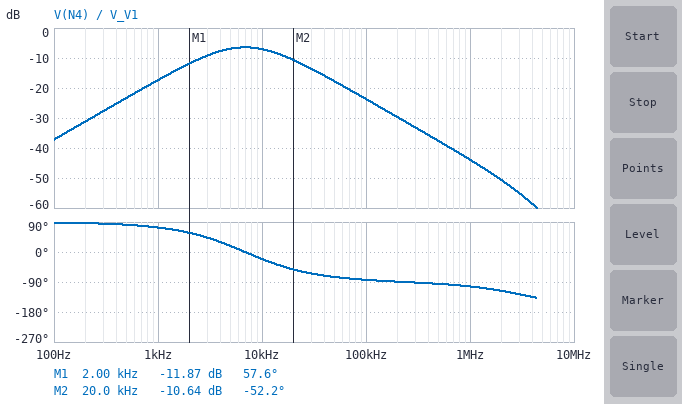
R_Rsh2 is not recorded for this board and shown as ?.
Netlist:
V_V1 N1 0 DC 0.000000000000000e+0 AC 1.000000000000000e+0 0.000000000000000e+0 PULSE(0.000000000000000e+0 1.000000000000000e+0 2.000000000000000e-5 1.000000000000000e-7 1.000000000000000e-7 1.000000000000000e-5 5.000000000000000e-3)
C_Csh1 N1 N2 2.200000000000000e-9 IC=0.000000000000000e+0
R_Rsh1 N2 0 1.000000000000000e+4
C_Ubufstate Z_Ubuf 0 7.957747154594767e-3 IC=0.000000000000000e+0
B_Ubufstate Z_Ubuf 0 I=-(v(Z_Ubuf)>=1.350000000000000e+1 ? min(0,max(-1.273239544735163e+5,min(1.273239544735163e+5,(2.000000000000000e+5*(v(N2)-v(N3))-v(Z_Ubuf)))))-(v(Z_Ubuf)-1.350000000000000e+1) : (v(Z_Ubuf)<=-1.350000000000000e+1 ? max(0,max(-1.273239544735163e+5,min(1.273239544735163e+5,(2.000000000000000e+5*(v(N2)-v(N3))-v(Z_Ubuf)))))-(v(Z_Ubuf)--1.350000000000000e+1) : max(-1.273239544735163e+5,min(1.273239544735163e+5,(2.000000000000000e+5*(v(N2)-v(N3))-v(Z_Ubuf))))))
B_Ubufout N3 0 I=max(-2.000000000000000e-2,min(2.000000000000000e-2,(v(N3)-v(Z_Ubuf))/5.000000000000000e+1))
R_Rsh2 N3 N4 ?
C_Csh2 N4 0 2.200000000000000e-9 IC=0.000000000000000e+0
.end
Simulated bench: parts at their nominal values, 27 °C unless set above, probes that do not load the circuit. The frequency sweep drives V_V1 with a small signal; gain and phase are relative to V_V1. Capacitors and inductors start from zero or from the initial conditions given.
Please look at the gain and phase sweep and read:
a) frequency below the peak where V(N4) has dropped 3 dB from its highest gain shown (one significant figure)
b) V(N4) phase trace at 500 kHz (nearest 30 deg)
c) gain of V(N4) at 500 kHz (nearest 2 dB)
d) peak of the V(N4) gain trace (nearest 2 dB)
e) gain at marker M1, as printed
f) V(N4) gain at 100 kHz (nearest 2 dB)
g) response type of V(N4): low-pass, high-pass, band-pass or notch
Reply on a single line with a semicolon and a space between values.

3 kHz; -90 deg; -38 dB; -6 dB; -11.87 dB; -24 dB; band-pass
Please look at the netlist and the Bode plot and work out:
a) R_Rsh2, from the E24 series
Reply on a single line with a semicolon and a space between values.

11 kΩ
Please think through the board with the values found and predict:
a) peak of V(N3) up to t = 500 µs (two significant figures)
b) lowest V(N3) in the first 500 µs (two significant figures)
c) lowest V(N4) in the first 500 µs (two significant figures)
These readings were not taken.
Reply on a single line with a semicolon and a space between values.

990 mV; -360 mV; -56 mV
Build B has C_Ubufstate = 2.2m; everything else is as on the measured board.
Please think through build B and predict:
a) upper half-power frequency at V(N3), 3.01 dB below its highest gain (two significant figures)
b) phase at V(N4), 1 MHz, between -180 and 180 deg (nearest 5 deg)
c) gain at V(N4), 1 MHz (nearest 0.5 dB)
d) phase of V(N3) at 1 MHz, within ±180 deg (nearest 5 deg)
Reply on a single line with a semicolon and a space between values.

14 MHz; -95 deg; -43.5 dB; -5 deg
